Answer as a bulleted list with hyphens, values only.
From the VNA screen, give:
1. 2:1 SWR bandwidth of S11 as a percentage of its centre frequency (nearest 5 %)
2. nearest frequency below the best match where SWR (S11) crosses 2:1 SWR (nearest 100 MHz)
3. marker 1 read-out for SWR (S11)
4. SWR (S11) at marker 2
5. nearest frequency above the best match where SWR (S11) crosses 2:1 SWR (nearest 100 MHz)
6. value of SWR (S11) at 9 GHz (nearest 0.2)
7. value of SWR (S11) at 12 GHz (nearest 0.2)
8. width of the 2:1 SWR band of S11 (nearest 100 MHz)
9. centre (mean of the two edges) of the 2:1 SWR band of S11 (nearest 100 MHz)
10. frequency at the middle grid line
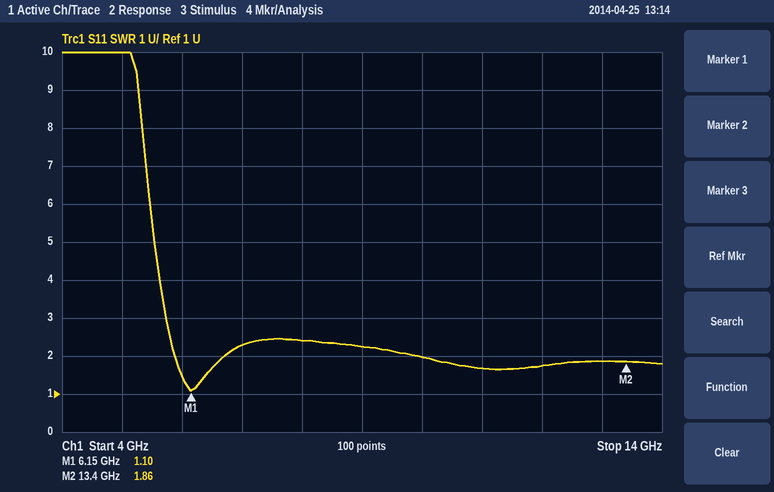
- 15 %
- 5.9 GHz
- 1.10
- 1.86
- 6.7 GHz
- 2.2
- 1.8
- 800 MHz
- 6.3 GHz
- 9 GHz
